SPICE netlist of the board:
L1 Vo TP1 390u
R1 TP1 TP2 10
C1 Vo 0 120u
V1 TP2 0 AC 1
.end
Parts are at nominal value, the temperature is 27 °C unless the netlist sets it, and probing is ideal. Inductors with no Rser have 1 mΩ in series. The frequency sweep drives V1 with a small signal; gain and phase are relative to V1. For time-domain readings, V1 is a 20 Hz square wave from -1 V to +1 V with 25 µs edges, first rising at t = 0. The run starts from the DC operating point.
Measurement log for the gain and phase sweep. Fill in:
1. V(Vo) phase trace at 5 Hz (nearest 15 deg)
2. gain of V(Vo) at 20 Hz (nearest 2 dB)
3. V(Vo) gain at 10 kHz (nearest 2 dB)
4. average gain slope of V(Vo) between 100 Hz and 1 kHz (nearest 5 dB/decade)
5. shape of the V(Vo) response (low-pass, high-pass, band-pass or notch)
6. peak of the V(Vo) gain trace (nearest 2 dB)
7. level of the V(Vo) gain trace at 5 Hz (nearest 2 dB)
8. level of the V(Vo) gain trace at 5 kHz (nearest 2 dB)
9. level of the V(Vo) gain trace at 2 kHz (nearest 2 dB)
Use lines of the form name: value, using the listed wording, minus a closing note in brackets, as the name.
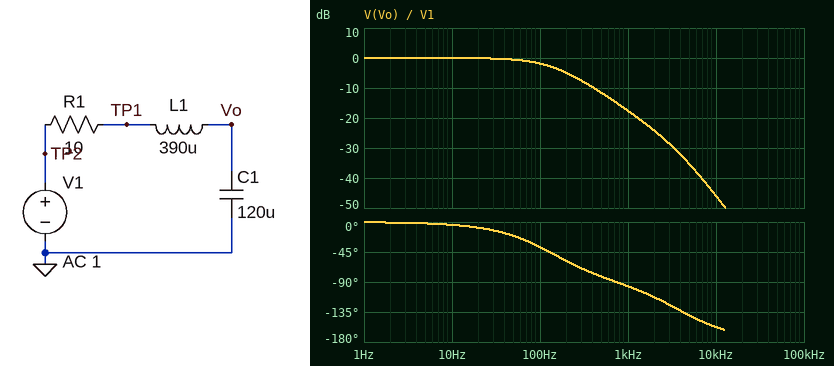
V(Vo) phase trace at 5 Hz: 0 deg
gain of V(Vo) at 20 Hz: 0 dB
V(Vo) gain at 10 kHz: -46 dB
average gain slope of V(Vo) between 100 Hz and 1 kHz: -15 dB/decade
shape of the V(Vo) response: low-pass
peak of the V(Vo) gain trace: 0 dB
level of the V(Vo) gain trace at 5 Hz: 0 dB
level of the V(Vo) gain trace at 5 kHz: -36 dB
level of the V(Vo) gain trace at 2 kHz: -24 dB
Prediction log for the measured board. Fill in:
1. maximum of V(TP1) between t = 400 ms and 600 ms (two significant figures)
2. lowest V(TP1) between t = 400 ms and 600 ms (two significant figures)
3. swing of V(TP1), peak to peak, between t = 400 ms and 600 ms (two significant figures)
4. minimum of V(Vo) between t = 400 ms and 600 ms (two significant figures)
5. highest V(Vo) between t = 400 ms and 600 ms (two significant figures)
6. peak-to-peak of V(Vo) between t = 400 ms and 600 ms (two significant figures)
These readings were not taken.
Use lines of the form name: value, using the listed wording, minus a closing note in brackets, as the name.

maximum of V(TP1) between t = 400 ms and 600 ms: 1.0 V
lowest V(TP1) between t = 400 ms and 600 ms: -1.0 V
swing of V(TP1), peak to peak, between t = 400 ms and 600 ms: 2.0 V
minimum of V(Vo) between t = 400 ms and 600 ms: -1.0 V
highest V(Vo) between t = 400 ms and 600 ms: 1.0 V
peak-to-peak of V(Vo) between t = 400 ms and 600 ms: 2.0 V
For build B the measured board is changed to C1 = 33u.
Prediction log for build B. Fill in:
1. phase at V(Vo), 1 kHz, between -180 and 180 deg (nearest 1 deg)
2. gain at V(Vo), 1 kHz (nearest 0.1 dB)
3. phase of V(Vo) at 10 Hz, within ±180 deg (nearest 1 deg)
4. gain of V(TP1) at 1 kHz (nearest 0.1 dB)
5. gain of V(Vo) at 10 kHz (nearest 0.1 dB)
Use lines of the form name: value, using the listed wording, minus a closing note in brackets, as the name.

phase at V(Vo), 1 kHz, between -180 and 180 deg: -77 deg
gain at V(Vo), 1 kHz: -6.6 dB
phase of V(Vo) at 10 Hz, within ±180 deg: -1 deg
gain of V(TP1) at 1 kHz: -12.7 dB
gain of V(Vo) at 10 kHz: -34.6 dB
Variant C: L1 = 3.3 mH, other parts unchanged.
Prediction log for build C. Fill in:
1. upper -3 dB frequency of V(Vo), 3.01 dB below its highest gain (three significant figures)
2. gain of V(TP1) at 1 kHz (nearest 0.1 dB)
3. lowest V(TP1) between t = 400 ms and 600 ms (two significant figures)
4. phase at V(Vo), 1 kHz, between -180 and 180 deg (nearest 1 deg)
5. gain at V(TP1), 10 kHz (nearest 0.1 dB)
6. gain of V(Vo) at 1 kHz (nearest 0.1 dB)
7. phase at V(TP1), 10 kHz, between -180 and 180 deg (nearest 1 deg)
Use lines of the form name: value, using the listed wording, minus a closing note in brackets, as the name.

upper -3 dB frequency of V(Vo), 3.01 dB below its highest gain: 174 Hz
gain of V(TP1) at 1 kHz: -1.0 dB
lowest V(TP1) between t = 400 ms and 600 ms: -1.0 V
phase at V(Vo), 1 kHz, between -180 and 180 deg: -153 deg
gain at V(TP1), 10 kHz: 0 dB
gain of V(Vo) at 1 kHz: -24.3 dB
phase at V(TP1), 10 kHz, between -180 and 180 deg: 3 deg
